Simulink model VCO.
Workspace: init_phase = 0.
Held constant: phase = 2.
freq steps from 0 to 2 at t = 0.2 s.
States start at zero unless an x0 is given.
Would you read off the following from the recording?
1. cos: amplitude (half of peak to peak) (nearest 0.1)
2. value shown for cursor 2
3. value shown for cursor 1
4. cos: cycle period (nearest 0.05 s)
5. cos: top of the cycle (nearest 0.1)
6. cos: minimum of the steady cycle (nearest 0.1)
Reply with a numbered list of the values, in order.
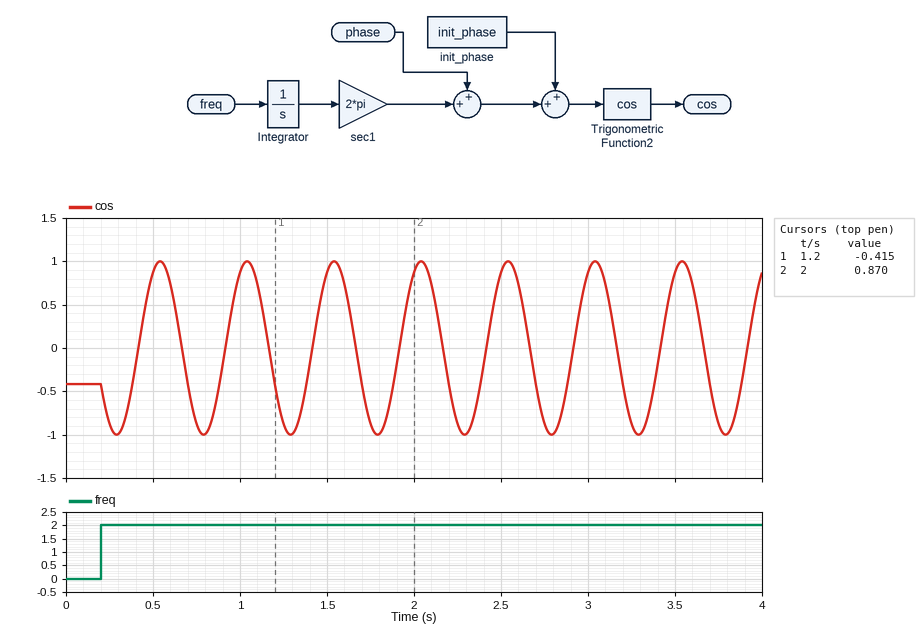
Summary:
1. 1.0
2. 0.870
3. -0.415
4. 0.50 s
5. 1.0
6. -1.0
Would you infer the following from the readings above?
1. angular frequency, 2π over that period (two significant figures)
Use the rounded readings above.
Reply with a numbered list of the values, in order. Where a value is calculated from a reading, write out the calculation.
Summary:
1. 2π / 0.5 = 13 rad/s
